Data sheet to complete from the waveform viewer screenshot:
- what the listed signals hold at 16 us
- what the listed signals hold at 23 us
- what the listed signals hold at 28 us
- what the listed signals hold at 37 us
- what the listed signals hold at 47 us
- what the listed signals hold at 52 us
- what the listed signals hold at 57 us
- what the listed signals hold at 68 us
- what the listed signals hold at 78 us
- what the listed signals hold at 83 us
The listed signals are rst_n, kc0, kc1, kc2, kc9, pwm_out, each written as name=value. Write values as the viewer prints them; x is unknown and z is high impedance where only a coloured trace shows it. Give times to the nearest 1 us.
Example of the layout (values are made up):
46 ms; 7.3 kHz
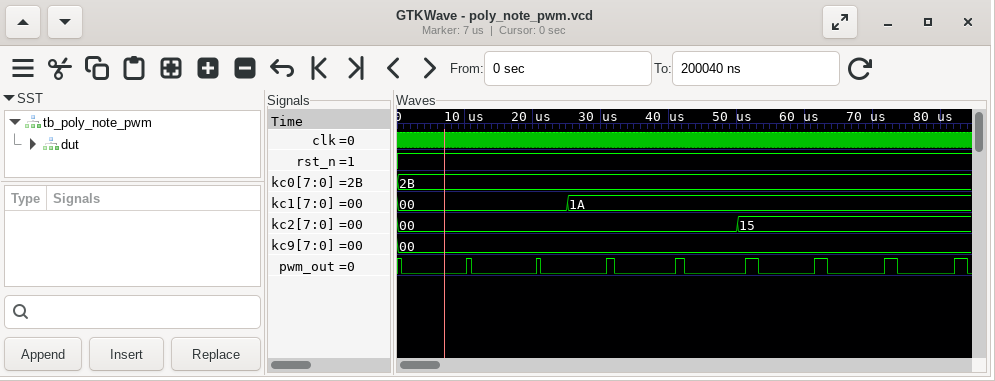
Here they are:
rst_n=1, kc0=2B, kc1=00, kc2=00, kc9=00, pwm_out=0; rst_n=1, kc0=2B, kc1=00, kc2=00, kc9=00, pwm_out=0; rst_n=1, kc0=2B, kc1=1A, kc2=00, kc9=00, pwm_out=0; rst_n=1, kc0=2B, kc1=1A, kc2=00, kc9=00, pwm_out=0; rst_n=1, kc0=2B, kc1=1A, kc2=00, kc9=00, pwm_out=0; rst_n=1, kc0=2B, kc1=1A, kc2=15, kc9=00, pwm_out=1; rst_n=1, kc0=2B, kc1=1A, kc2=15, kc9=00, pwm_out=0; rst_n=1, kc0=2B, kc1=1A, kc2=15, kc9=00, pwm_out=0; rst_n=1, kc0=2B, kc1=1A, kc2=15, kc9=00, pwm_out=0; rst_n=1, kc0=2B, kc1=1A, kc2=15, kc9=00, pwm_out=1
